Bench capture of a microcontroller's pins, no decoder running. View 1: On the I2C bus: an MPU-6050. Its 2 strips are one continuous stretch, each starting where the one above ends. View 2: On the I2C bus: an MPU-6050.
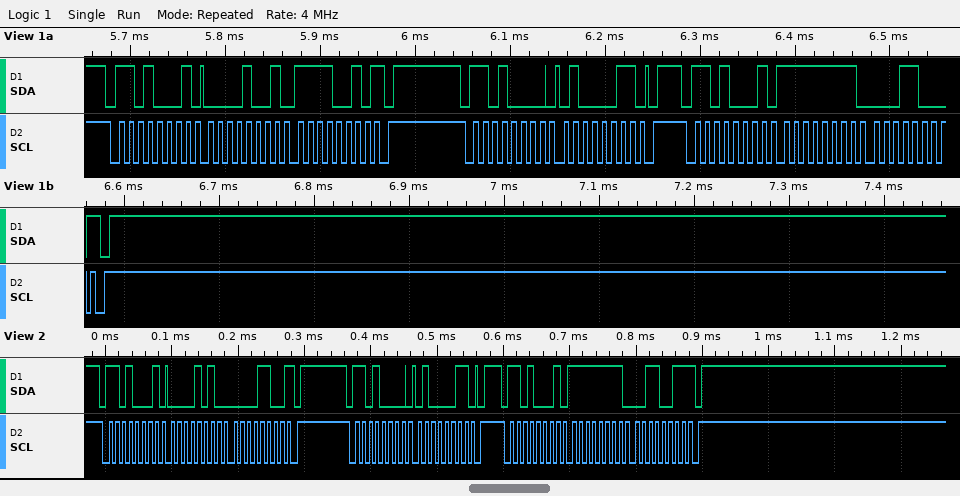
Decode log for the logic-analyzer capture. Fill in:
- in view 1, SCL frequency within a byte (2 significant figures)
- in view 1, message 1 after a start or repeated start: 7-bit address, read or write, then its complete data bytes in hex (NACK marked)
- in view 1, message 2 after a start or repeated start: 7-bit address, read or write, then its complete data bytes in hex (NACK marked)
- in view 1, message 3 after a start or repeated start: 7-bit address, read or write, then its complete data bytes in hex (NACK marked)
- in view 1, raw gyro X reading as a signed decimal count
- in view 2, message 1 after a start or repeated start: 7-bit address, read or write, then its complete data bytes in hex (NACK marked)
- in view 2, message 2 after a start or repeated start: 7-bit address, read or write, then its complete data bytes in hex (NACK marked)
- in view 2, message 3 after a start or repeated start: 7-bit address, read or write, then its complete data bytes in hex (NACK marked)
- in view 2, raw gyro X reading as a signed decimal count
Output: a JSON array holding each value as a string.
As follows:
["100 kHz", "0x68 read: 09 F2 NACK", "0x68 write: 43", "0x68 read: FF 18 NACK", "-232", "0x68 read: 0A 0C NACK", "0x68 write: 43", "0x68 read: FF 33 NACK", "-205"]
